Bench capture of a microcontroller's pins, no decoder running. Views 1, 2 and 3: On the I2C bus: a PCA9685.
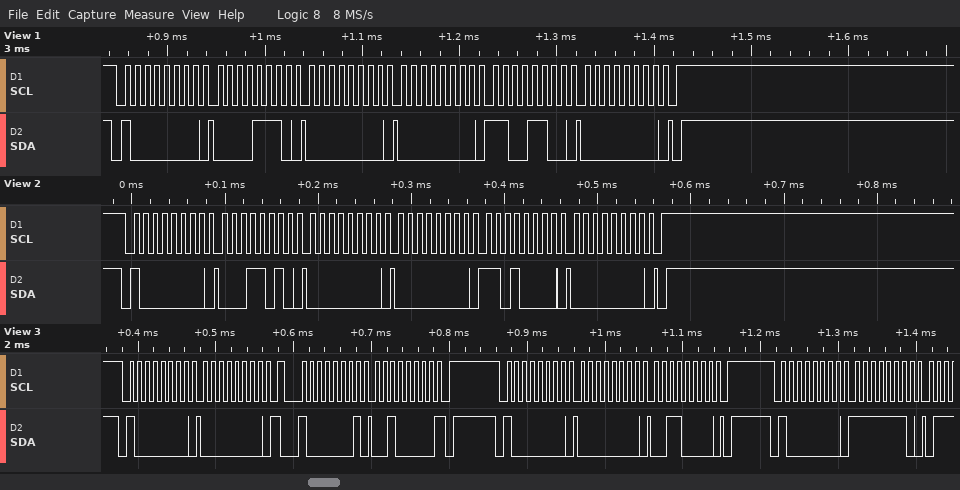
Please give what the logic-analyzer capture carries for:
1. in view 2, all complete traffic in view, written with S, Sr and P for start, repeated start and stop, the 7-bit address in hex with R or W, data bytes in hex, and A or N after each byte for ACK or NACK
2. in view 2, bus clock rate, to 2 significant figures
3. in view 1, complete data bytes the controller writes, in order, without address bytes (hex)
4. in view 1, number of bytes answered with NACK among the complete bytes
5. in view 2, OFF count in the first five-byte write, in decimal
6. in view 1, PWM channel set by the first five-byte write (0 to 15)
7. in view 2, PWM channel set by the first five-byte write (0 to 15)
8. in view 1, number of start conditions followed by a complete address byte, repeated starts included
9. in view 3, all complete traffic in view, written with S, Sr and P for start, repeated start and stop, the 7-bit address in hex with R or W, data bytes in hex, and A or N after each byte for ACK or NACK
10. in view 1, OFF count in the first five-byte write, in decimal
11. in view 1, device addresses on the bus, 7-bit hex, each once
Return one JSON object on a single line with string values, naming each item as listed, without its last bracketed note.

{"in view 2, all complete traffic in view, written with S, Sr and P for start, repeated start and stop, the 7-bit address in hex with R or W, data bytes in hex, and A or N after each byte for ACK or NACK": "S 40W A 1A A 00 A 00 A D0 A 00 A P", "in view 2, bus clock rate, to 2 significant figures": "100 kHz", "in view 1, complete data bytes the controller writes, in order, without address bytes": "0E 00 00 CC 00", "in view 1, number of bytes answered with NACK among the complete bytes": "0", "in view 2, OFF count in the first five-byte write, in decimal": "208", "in view 1, PWM channel set by the first five-byte write": "2", "in view 2, PWM channel set by the first five-byte write": "5", "in view 1, number of start conditions followed by a complete address byte, repeated starts included": "1", "in view 3, all complete traffic in view, written with S, Sr and P for start, repeated start and stop, the 7-bit address in hex with R or W, data bytes in hex, and A or N after each byte for ACK or NACK": "S 40W A 00 A Sr 40R A 20 N P S 40W A 00 A 30 A P S 40W A FE A", "in view 1, OFF count in the first five-byte write, in decimal": "204", "in view 1, device addresses on the bus, 7-bit hex, each once": "0x40"}
